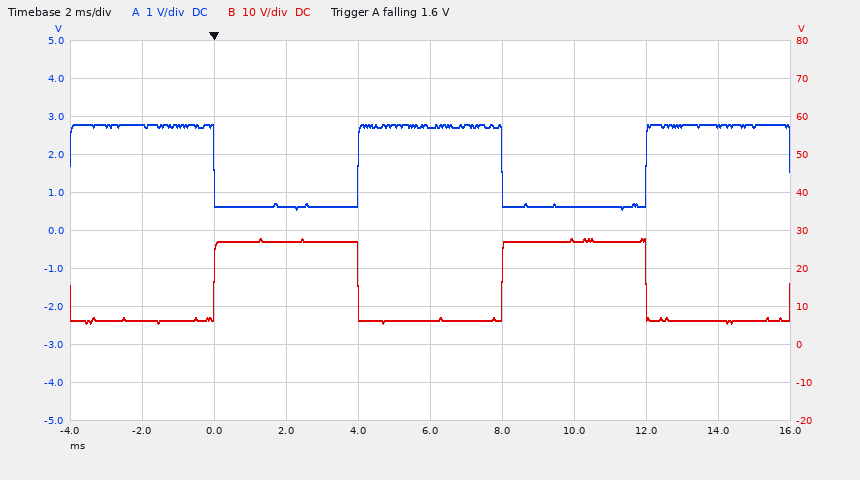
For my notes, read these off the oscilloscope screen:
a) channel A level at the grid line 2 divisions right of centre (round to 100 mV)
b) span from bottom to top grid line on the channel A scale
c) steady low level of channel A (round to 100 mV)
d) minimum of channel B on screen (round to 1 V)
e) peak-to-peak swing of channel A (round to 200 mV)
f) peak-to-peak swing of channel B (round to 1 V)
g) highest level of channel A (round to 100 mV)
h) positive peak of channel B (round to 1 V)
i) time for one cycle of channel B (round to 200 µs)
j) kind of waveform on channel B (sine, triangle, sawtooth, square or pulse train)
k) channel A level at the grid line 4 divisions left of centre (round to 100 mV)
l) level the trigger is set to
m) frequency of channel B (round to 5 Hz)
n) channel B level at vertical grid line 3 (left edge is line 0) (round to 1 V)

600 mV
10 V
600 mV
6 V
2.2 V
22 V
2.8 V
28 V
8.0 ms
square
2.8 V
1.6 V
125 Hz
27 V
